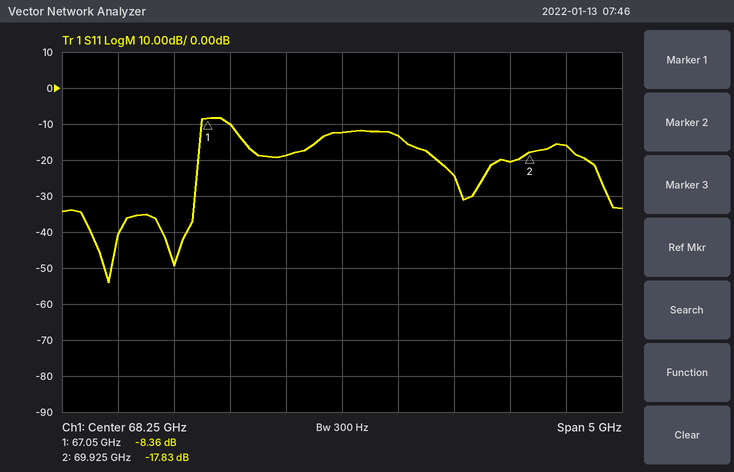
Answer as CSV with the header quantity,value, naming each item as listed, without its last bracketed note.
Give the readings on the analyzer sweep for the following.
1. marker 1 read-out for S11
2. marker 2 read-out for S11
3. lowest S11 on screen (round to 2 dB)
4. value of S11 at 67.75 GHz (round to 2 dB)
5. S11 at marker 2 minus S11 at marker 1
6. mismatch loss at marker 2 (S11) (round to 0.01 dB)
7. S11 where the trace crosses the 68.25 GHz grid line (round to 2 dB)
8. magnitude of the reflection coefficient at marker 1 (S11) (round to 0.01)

quantity,value
marker 1 read-out for S11,-8.36 dB
marker 2 read-out for S11,-17.83 dB
lowest S11 on screen,-54 dB
value of S11 at 67.75 GHz,-18 dB
S11 at marker 2 minus S11 at marker 1,-9.47 dB
mismatch loss at marker 2 (S11),0.07 dB
S11 where the trace crosses the 68.25 GHz grid line,-12 dB
magnitude of the reflection coefficient at marker 1 (S11),0.38
